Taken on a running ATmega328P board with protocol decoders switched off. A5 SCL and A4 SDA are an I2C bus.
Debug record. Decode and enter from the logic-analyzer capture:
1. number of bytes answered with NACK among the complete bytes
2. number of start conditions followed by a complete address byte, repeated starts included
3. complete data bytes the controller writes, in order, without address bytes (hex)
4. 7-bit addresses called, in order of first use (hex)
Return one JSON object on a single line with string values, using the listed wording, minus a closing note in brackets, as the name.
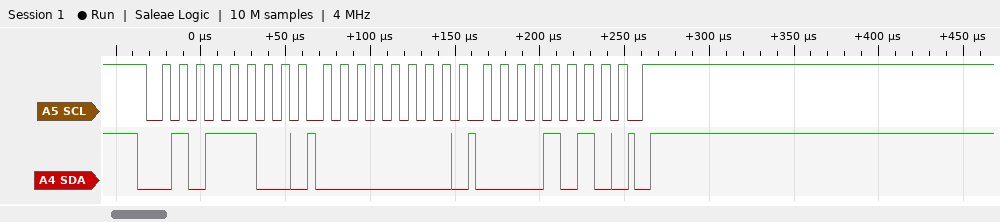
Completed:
{"number of bytes answered with NACK among the complete bytes": "0", "number of start conditions followed by a complete address byte, repeated starts included": "1", "complete data bytes the controller writes, in order, without address bytes": "00 0A", "7-bit addresses called, in order of first use": "0x2E"}
